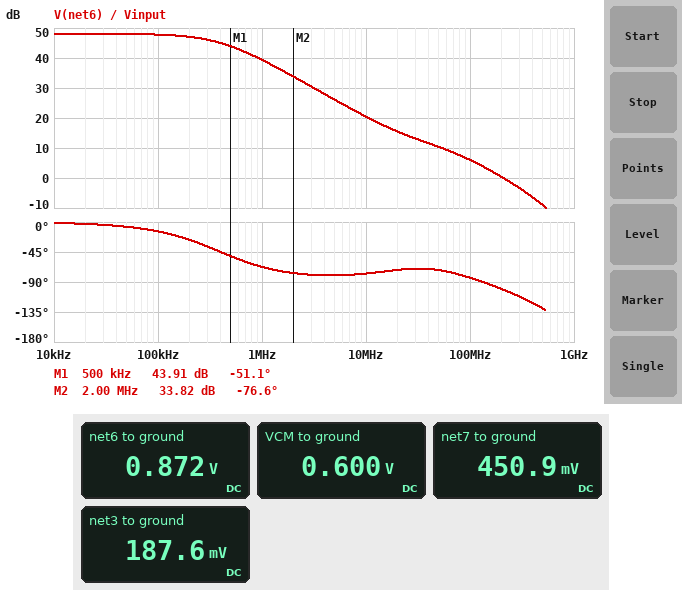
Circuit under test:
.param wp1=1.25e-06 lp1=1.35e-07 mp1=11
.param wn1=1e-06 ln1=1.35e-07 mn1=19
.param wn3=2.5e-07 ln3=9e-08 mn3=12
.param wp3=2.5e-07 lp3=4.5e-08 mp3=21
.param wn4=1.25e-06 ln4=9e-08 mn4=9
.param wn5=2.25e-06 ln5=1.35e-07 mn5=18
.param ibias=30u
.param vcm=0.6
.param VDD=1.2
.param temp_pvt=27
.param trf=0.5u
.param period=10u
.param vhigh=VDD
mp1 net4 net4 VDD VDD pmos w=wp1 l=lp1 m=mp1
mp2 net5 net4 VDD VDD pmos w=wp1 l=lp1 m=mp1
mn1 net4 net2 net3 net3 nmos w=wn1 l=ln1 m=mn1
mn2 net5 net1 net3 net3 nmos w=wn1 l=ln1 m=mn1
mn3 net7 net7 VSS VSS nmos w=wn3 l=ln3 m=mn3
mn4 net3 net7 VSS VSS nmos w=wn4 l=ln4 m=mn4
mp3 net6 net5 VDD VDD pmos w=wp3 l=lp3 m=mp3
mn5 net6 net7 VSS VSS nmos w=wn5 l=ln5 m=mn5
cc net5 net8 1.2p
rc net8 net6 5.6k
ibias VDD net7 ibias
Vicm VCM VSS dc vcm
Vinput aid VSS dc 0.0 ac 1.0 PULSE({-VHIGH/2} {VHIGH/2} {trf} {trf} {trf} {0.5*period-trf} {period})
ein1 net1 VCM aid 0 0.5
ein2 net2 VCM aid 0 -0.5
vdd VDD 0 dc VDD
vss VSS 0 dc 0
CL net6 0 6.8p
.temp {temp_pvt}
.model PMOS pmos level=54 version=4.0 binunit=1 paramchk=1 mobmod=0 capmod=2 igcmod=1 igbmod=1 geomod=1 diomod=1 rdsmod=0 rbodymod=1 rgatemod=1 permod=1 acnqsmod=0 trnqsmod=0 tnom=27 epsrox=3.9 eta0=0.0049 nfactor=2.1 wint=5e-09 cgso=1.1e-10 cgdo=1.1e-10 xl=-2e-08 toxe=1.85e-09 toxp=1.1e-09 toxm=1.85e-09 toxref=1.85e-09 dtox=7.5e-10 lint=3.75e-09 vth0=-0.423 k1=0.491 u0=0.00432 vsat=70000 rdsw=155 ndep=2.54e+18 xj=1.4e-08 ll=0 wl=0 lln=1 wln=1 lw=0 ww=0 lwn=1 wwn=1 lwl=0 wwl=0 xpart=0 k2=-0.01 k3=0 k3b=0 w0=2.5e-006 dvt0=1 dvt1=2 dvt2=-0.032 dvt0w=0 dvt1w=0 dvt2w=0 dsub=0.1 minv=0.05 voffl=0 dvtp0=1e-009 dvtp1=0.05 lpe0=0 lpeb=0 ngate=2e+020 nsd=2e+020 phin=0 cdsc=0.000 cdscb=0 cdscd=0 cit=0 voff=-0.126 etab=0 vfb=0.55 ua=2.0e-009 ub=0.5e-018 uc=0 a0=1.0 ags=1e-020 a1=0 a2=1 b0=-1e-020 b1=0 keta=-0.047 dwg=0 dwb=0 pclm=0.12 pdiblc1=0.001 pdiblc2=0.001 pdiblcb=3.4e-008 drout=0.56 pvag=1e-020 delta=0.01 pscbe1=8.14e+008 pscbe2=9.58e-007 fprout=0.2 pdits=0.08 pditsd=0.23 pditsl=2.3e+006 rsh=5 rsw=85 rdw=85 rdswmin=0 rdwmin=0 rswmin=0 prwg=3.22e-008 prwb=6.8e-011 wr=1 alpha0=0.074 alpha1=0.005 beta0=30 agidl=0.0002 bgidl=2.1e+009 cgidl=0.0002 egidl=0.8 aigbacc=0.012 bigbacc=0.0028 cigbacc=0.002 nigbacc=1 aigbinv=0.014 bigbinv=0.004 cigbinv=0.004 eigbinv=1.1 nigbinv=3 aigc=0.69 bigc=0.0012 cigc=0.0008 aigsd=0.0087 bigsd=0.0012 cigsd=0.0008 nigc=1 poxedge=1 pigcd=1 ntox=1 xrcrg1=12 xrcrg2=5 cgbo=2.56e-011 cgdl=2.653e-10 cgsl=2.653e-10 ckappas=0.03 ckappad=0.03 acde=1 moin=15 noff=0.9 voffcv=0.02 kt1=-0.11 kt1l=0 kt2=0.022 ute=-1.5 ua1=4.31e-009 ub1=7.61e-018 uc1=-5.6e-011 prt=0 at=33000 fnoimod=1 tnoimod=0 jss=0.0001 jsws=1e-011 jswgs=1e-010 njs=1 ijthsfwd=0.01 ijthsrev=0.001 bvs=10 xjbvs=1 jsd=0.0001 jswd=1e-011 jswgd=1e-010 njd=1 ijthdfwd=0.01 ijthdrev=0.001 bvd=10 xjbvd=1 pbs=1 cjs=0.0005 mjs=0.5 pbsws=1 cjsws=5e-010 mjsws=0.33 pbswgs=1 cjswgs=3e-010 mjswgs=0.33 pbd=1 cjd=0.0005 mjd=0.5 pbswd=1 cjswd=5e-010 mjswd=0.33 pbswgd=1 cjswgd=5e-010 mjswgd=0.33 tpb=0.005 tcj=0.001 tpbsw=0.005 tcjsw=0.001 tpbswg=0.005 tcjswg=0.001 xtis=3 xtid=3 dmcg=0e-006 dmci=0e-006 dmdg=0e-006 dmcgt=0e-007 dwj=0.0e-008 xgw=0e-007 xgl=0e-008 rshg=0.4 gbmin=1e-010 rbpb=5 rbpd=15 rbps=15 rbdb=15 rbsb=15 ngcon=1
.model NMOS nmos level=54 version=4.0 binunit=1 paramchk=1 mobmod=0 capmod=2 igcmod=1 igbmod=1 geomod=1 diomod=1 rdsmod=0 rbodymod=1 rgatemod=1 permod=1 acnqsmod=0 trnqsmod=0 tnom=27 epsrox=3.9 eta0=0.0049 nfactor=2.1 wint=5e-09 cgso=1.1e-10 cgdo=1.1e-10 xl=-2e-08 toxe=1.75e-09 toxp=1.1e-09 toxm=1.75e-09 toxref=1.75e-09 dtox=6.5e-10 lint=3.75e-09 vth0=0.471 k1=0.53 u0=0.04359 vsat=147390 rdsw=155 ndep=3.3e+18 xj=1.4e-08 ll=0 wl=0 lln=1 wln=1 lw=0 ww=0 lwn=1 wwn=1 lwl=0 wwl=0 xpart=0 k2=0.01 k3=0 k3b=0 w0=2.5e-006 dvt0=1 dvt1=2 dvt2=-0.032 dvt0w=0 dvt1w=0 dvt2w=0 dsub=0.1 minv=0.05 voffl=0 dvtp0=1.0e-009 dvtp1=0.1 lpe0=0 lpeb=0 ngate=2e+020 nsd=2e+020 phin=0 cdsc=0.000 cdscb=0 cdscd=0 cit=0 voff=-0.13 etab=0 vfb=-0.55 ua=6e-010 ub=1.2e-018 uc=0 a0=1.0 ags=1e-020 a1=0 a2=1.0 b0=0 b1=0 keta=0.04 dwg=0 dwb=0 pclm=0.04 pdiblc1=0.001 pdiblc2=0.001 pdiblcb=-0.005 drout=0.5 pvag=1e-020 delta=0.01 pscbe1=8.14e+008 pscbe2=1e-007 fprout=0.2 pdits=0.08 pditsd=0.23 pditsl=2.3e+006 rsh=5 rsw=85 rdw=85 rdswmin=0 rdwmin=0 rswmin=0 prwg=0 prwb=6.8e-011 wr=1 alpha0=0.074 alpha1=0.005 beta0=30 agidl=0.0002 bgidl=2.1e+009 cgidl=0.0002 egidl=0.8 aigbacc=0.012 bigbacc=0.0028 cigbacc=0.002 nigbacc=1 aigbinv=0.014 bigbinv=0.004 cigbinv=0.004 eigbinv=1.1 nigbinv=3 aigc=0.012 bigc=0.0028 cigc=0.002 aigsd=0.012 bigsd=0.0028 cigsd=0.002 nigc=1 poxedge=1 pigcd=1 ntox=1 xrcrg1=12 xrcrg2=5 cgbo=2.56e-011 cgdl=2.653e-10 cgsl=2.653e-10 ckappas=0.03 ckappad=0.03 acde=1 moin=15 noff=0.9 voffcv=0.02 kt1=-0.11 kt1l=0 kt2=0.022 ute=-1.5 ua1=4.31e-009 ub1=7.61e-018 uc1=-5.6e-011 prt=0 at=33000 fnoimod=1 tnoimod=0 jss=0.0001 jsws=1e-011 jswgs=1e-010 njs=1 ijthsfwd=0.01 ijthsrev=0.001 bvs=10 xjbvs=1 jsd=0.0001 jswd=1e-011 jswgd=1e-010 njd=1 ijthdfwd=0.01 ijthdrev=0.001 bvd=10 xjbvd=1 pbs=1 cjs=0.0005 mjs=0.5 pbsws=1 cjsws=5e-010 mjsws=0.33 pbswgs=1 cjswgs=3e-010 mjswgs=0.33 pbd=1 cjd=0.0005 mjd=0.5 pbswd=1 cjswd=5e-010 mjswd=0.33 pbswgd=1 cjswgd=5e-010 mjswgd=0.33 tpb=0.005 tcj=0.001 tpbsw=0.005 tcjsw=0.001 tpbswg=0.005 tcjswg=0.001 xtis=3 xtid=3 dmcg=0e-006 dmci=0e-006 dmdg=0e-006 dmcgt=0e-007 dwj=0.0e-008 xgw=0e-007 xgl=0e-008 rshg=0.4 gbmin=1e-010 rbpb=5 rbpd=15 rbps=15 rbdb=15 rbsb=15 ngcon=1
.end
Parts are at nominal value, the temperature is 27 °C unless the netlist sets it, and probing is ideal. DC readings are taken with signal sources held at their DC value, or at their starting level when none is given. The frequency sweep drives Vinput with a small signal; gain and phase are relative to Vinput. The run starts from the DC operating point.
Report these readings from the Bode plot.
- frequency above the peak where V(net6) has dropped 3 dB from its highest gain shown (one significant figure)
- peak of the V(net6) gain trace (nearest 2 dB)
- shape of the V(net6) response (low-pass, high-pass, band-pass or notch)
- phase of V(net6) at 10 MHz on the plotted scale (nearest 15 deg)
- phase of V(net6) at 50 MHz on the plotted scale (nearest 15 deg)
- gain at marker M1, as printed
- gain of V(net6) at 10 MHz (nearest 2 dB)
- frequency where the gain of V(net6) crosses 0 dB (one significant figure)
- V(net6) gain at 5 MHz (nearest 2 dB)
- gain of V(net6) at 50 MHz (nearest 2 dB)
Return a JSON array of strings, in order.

["400 kHz", "48 dB", "low-pass", "-75 deg", "-75 deg", "43.91 dB", "20 dB", "200 MHz", "26 dB", "10 dB"]
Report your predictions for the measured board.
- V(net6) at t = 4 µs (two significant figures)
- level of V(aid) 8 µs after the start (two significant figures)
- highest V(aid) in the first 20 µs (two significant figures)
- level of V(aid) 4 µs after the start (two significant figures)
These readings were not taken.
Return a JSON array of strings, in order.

["1.2 V", "-600 mV", "600 mV", "600 mV"]
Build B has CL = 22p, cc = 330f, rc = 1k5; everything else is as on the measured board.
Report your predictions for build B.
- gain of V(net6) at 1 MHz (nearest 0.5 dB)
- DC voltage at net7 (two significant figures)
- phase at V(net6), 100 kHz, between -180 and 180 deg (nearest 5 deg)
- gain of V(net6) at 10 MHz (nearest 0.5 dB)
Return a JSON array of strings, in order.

["45.5 dB", "450 mV", "-5 deg", "28.0 dB"]
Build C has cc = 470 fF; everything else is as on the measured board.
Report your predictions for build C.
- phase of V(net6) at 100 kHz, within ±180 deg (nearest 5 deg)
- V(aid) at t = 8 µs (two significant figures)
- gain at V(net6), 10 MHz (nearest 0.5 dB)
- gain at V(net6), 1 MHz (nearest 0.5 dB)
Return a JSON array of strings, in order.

["-5 deg", "-600 mV", "27.5 dB", "45.0 dB"]
